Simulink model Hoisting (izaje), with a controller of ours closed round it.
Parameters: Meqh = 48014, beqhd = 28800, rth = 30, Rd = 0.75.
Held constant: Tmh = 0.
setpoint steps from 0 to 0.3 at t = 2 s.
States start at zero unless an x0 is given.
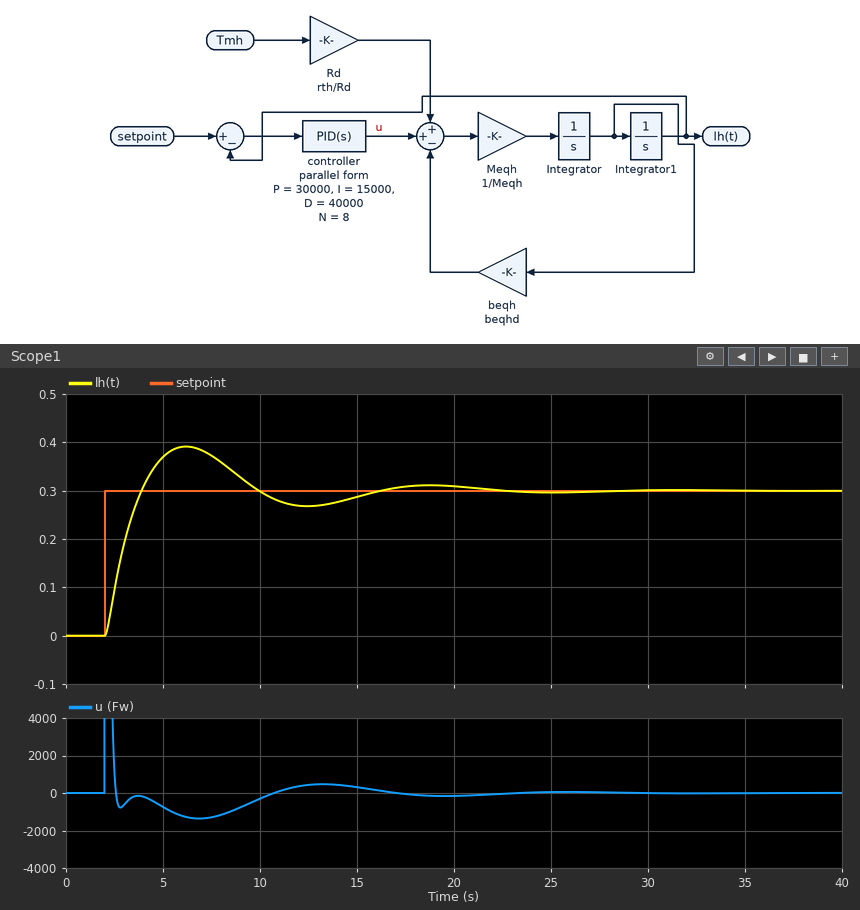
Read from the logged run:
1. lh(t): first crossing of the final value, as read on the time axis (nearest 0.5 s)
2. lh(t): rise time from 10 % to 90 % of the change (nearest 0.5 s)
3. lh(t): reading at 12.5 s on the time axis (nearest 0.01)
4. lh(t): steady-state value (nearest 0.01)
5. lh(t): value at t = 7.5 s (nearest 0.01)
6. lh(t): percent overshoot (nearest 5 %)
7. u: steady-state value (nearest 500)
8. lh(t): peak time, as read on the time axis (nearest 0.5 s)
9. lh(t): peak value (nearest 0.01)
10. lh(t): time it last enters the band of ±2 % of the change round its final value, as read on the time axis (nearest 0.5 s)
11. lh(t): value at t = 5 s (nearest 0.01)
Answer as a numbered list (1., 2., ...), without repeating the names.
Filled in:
1. 4.0 s
2. 1.5 s
3. 0.27
4. 0.30
5. 0.37
6. 30 %
7. 0
8. 6.0 s
9. 0.39
10. 21.0 s
11. 0.37
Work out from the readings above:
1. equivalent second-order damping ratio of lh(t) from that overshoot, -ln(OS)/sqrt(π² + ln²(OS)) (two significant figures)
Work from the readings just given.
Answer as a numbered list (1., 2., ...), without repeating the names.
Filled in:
1. 0.36
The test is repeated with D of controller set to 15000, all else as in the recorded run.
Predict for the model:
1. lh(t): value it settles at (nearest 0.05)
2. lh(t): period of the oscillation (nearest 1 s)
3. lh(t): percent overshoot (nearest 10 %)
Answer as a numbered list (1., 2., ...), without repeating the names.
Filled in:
1. 0.30
2. 9 s
3. 60 %
